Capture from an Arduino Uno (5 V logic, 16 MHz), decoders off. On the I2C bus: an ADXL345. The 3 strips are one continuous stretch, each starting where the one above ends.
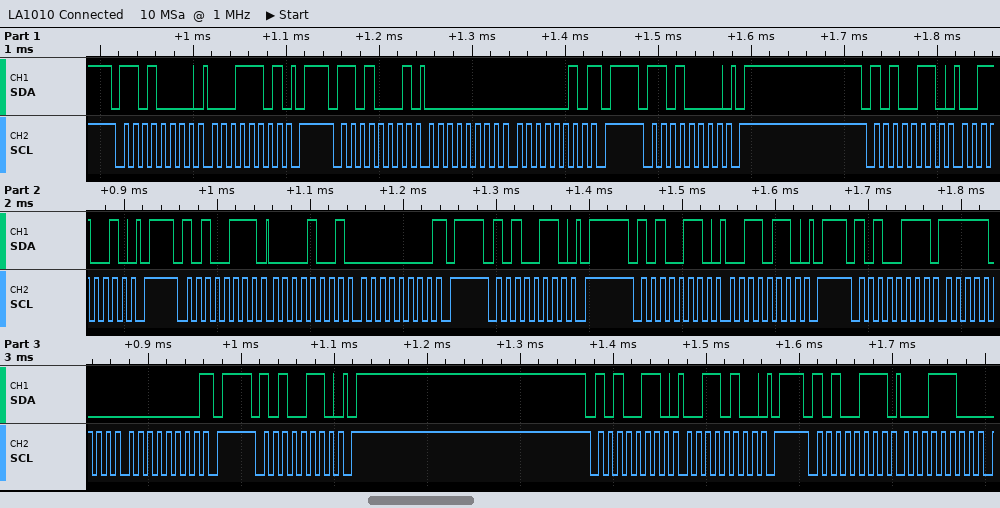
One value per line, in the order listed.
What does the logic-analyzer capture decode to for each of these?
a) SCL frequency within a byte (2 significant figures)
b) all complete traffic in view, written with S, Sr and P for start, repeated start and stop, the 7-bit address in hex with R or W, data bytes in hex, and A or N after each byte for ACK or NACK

100 kHz
S 68W A 1D A P S 68R A 00 A 02 N P S 68W A P S 53W A 32 A P S 53R A 09 A 00 N P S 53W A P S 53W A 36 A P S 53R A F8 A 00 N P S 53W A P S 53W A 34 A P S 53R A 1C A
